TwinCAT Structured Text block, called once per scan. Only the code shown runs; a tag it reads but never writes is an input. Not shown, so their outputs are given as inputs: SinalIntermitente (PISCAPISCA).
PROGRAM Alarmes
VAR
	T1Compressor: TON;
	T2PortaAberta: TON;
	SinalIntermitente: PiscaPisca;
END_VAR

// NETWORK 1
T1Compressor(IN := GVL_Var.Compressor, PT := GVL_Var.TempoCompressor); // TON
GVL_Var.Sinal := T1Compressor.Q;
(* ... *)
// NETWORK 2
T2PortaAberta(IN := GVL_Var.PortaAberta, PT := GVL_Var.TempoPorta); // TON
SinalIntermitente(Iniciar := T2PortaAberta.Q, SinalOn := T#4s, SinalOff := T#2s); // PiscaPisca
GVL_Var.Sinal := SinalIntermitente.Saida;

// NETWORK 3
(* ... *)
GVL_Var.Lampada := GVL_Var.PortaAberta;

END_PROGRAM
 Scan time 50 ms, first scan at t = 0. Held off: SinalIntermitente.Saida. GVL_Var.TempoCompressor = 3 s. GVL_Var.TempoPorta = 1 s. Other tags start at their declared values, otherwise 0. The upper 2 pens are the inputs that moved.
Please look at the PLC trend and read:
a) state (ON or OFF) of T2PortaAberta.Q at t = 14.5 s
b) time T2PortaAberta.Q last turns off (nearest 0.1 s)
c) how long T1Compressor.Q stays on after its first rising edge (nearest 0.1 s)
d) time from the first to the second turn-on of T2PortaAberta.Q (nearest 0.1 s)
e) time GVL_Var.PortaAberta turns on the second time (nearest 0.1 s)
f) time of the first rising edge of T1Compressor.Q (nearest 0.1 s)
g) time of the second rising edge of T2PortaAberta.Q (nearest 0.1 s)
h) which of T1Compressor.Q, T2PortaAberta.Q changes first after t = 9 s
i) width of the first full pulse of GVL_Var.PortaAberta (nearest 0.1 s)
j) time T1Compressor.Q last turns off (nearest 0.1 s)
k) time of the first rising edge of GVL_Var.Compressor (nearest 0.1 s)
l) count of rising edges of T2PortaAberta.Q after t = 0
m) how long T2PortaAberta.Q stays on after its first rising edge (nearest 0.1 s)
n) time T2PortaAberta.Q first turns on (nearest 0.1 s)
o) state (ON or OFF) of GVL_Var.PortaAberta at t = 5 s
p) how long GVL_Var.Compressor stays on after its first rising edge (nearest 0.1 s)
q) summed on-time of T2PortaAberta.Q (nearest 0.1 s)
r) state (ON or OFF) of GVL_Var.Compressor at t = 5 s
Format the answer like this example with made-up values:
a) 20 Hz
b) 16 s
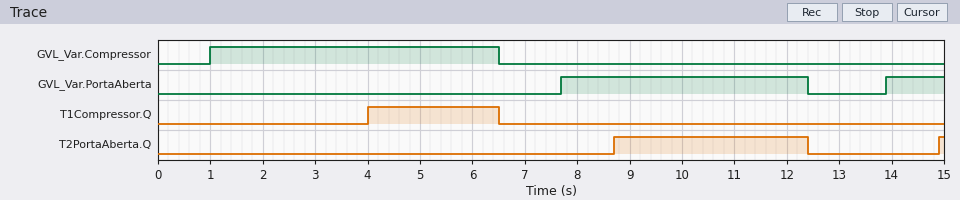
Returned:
a) OFF
b) 12.4 s
c) 2.5 s
d) 6.2 s
e) 13.9 s
f) 4.0 s
g) 14.9 s
h) T2PortaAberta.Q
i) 4.7 s
j) 6.5 s
k) 1.0 s
l) 2
m) 3.7 s
n) 8.7 s
o) OFF
p) 5.5 s
q) 3.8 s
r) ON
